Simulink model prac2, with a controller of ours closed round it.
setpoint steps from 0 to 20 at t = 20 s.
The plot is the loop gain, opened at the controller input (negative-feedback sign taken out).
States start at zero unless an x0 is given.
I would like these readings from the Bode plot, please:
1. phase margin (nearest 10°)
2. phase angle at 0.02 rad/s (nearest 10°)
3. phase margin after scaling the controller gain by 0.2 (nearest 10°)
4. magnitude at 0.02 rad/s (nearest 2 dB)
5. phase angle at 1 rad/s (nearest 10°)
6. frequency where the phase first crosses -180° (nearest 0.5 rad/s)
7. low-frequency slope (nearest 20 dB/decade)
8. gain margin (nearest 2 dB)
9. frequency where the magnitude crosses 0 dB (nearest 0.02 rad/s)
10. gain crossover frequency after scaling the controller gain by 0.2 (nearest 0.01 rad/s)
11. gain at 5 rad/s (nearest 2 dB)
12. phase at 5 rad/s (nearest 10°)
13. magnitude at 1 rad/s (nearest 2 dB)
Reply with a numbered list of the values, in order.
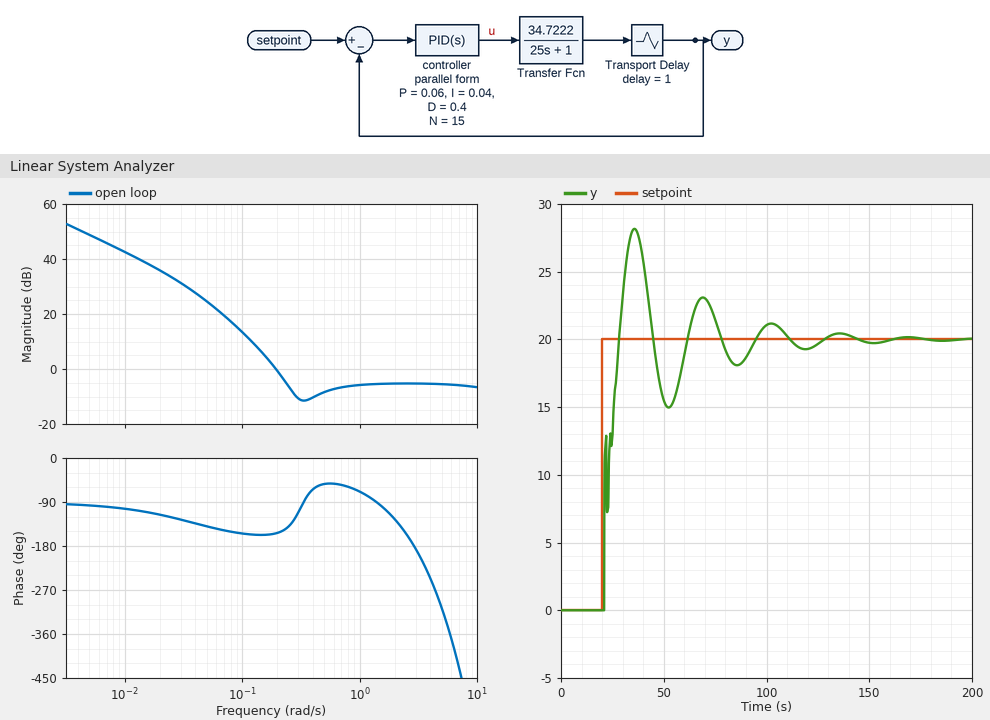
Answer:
1. 30°
2. -120°
3. 30°
4. 36 dB
5. -70°
6. 3.0 rad/s
7. -20 dB/decade
8. 6 dB
9. 0.20 rad/s
10. 0.10 rad/s
11. -6 dB
12. -310°
13. -6 dB
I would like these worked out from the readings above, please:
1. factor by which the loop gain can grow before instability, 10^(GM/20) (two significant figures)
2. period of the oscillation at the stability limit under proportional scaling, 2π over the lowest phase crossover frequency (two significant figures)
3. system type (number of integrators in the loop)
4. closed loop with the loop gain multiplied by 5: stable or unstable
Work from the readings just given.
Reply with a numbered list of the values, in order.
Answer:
1. 2.0
2. 2.1 s
3. 1
4. unstable
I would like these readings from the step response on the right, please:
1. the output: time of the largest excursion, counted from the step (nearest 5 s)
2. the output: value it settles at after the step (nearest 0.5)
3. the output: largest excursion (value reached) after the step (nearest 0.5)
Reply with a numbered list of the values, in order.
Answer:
1. 15 s
2. 20.0
3. 28.0
